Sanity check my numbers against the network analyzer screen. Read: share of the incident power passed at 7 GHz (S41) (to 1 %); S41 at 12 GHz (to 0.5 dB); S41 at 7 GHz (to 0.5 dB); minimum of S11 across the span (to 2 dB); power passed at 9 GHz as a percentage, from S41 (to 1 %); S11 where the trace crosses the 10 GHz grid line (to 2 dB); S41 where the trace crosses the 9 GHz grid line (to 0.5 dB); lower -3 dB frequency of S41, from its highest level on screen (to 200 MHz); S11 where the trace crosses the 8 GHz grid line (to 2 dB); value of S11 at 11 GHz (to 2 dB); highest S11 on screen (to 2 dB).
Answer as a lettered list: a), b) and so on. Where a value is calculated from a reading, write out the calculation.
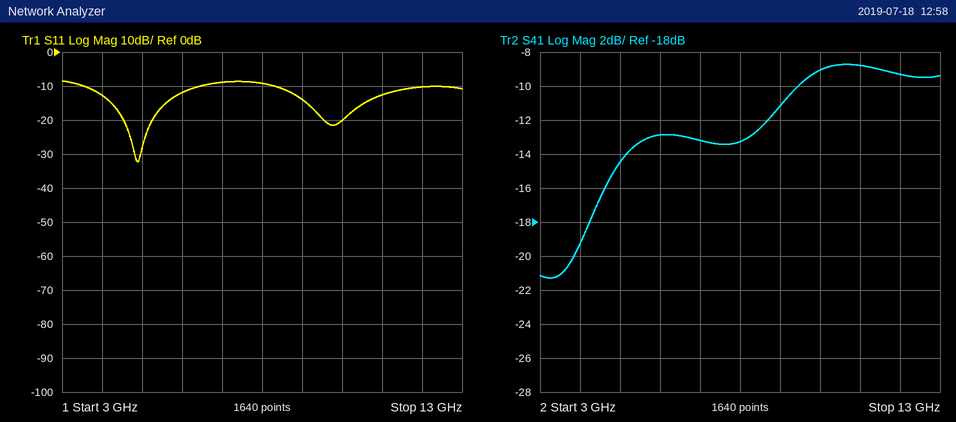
a) 10^(-13/10) ≈ 5 %
b) -9.5 dB
c) -13.0 dB
d) -32 dB
e) 10^(-11/10) ≈ 8 %
f) -20 dB
g) -11.0 dB
h) 8.8 GHz
i) -10 dB
j) -12 dB
k) -8 dB
